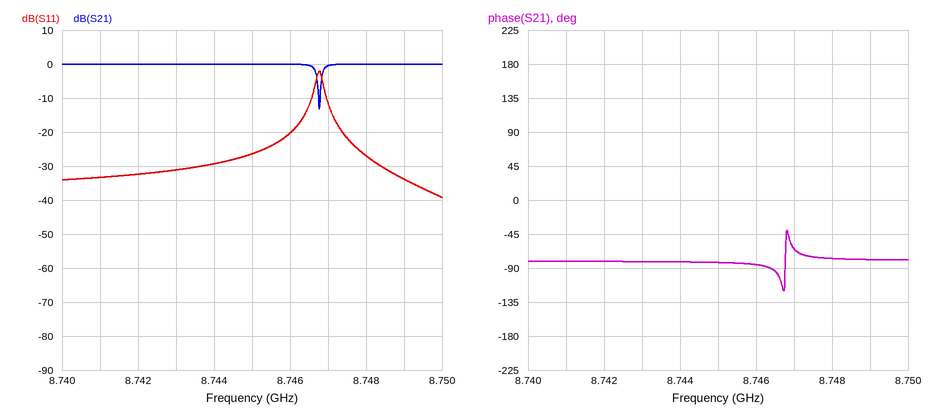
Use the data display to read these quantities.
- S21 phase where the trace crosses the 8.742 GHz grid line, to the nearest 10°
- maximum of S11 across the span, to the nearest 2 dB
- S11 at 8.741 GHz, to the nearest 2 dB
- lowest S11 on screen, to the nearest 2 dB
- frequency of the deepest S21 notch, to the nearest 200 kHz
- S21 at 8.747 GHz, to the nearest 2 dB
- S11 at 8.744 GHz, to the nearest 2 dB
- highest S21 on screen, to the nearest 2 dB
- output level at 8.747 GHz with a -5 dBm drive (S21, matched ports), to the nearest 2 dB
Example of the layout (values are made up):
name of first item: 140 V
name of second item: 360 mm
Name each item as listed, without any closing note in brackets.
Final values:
S21 phase where the trace crosses the 8.742 GHz grid line, to the nearest 10°: -80°
maximum of S11 across the span, to the nearest 2 dB: -2 dB
S11 at 8.741 GHz, to the nearest 2 dB: -34 dB
lowest S11 on screen, to the nearest 2 dB: -40 dB
frequency of the deepest S21 notch, to the nearest 200 kHz: 8.7468 GHz
S21 at 8.747 GHz, to the nearest 2 dB: 0 dB
S11 at 8.744 GHz, to the nearest 2 dB: -30 dB
highest S21 on screen, to the nearest 2 dB: 0 dB
output level at 8.747 GHz with a -5 dBm drive (S21, matched ports), to the nearest 2 dB: -6 dBm
